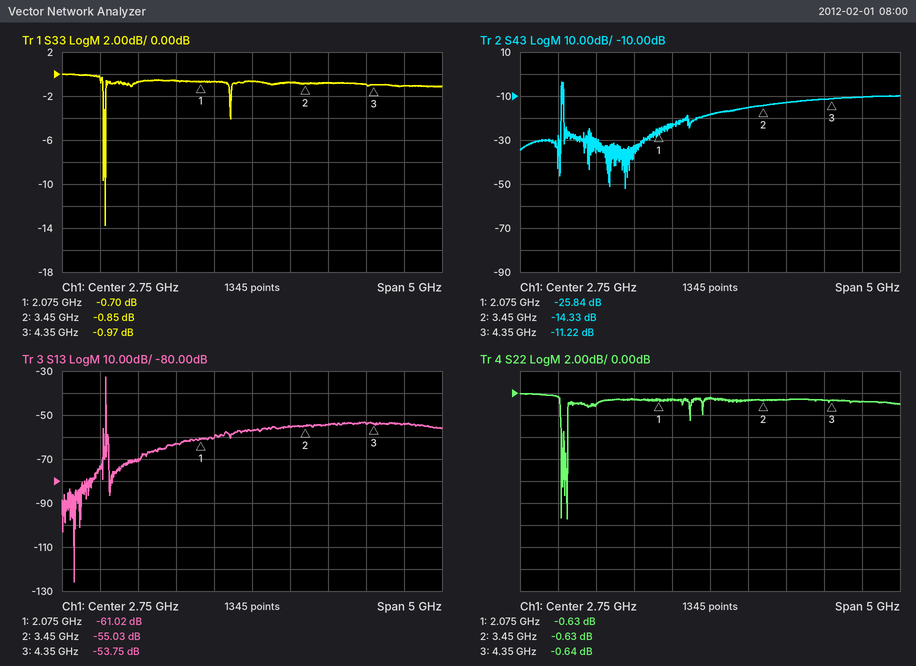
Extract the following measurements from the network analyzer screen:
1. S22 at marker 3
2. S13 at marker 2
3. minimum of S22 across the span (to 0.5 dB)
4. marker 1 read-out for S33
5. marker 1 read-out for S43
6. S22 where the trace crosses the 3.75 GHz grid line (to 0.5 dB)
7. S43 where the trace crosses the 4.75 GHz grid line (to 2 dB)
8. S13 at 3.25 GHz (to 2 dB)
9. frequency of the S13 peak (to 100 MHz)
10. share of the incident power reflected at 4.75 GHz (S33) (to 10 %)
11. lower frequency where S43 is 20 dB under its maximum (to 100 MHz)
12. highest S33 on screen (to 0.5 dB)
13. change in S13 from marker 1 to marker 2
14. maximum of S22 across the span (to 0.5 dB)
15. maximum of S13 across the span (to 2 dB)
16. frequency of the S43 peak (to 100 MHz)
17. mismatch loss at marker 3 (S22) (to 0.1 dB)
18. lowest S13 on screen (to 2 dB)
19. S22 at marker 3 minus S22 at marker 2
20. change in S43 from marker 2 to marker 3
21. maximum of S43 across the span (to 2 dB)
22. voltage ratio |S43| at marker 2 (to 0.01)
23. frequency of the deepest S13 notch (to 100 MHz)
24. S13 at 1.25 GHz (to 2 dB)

-0.64 dB
-55.03 dB
-11.5 dB
-0.70 dB
-25.84 dB
-0.5 dB
-10 dB
-56 dB
800 MHz
80 %
800 MHz
0.0 dB
5.99 dB
0.0 dB
-32 dB
800 MHz
8.6 dB
-126 dB
-0.01 dB
3.11 dB
-4 dB
0.19
400 MHz
-70 dB
